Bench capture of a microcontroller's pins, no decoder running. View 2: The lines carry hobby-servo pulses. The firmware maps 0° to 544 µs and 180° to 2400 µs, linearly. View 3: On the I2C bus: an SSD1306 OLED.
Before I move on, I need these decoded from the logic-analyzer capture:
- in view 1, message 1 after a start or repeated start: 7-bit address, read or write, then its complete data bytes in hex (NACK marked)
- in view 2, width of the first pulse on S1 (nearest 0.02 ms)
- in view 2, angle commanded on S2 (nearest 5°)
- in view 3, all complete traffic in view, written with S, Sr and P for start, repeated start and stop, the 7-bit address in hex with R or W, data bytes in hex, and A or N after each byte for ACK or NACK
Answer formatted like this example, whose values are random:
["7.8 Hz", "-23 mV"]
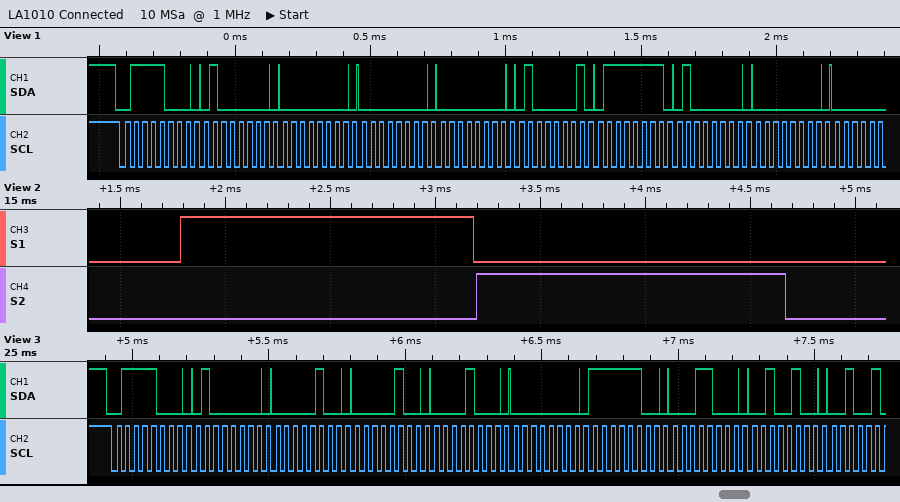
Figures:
["0x3C write: 40 00 00 00 41 7F 40 00", "1.40 ms", "90°", "S 3CW A 40 A 04 A 04 A 08 A 00 A FC A 18 A 24 A"]
